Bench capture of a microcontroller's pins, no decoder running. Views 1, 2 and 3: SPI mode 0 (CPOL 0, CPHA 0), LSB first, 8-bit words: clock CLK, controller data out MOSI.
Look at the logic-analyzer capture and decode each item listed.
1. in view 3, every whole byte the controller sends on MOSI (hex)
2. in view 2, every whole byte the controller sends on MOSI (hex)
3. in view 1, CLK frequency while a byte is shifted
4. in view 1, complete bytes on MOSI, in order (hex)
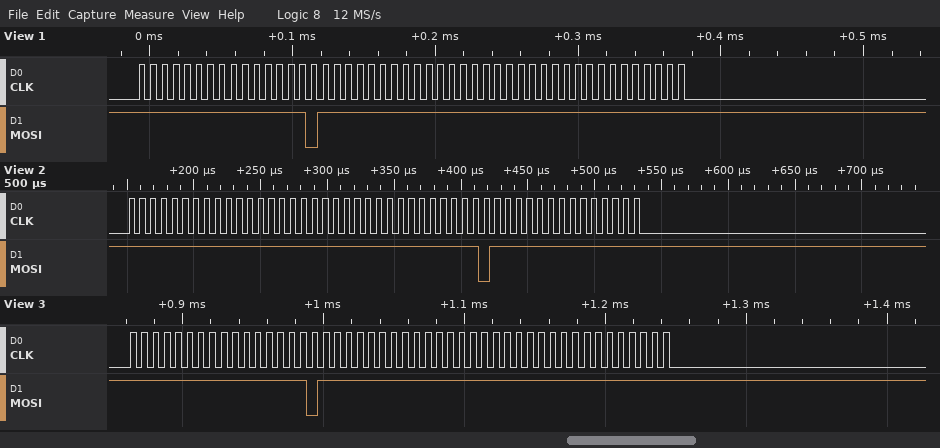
FF FF FE FF FF FF
FF FF FF FF FD FF
125 kHz
FF 7F FF FF FF FF
